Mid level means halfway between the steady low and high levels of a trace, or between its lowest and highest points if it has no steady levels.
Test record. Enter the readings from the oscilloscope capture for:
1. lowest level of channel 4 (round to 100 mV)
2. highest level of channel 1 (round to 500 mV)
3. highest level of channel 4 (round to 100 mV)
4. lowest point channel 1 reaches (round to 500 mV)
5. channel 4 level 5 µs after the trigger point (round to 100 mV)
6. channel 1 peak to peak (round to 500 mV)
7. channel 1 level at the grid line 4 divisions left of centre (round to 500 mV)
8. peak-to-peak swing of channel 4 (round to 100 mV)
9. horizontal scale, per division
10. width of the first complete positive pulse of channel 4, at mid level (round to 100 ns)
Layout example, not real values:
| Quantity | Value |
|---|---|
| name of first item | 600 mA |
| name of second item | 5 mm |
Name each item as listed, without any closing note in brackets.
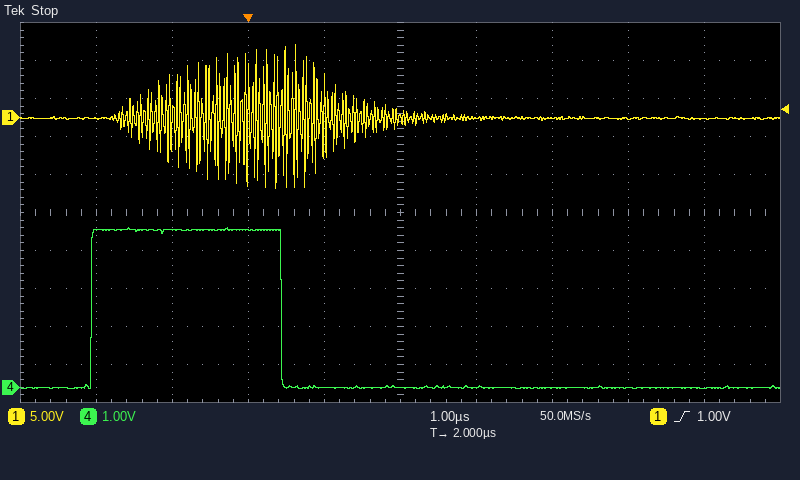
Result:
| Quantity | Value |
|---|---|
| lowest level of channel 4 | 0.0 V |
| highest level of channel 1 | 9.5 V |
| highest level of channel 4 | 4.2 V |
| lowest point channel 1 reaches | -9.5 V |
| channel 4 level 5 µs after the trigger point | 0.0 V |
| channel 1 peak to peak | 19.0 V |
| channel 1 level at the grid line 4 divisions left of centre | 0.0 V |
| peak-to-peak swing of channel 4 | 4.2 V |
| horizontal scale, per division | 1 µs |
| width of the first complete positive pulse of channel 4, at mid level | 2.5 µs |
